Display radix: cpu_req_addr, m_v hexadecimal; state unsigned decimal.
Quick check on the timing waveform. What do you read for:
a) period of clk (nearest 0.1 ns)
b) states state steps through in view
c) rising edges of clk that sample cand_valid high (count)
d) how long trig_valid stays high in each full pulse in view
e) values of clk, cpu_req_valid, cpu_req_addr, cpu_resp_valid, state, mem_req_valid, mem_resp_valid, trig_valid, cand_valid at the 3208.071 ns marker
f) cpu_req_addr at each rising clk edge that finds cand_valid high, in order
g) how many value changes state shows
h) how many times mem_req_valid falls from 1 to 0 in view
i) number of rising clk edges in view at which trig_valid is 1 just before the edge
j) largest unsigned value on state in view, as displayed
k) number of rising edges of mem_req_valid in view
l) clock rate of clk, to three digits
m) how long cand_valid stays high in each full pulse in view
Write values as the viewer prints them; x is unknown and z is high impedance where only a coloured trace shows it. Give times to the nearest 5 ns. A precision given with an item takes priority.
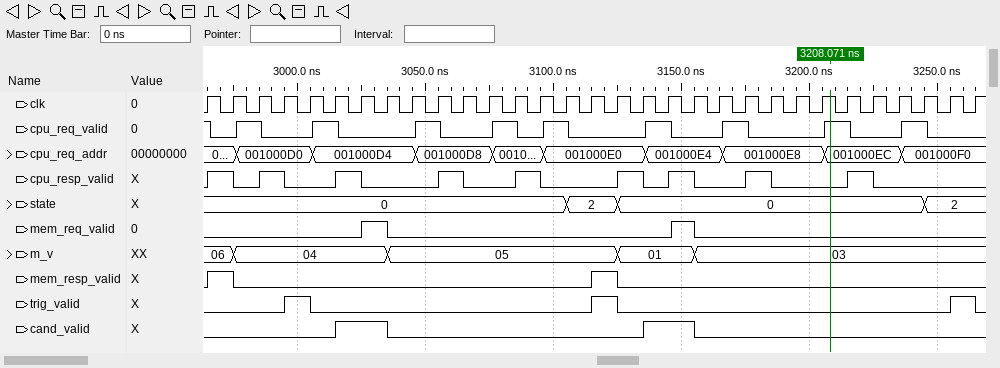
10 ns
0, 2, 0, 2
4
10 ns, 10 ns, 10 ns
clk=1, cpu_req_valid=1, cpu_req_addr=001000EC, cpu_resp_valid=0, state=0, mem_req_valid=0, mem_resp_valid=0, trig_valid=0, cand_valid=0
001000D4, 001000D4, 001000E4, 001000E4
3
2
3
2
2
100 MHz
20 ns, 20 ns
